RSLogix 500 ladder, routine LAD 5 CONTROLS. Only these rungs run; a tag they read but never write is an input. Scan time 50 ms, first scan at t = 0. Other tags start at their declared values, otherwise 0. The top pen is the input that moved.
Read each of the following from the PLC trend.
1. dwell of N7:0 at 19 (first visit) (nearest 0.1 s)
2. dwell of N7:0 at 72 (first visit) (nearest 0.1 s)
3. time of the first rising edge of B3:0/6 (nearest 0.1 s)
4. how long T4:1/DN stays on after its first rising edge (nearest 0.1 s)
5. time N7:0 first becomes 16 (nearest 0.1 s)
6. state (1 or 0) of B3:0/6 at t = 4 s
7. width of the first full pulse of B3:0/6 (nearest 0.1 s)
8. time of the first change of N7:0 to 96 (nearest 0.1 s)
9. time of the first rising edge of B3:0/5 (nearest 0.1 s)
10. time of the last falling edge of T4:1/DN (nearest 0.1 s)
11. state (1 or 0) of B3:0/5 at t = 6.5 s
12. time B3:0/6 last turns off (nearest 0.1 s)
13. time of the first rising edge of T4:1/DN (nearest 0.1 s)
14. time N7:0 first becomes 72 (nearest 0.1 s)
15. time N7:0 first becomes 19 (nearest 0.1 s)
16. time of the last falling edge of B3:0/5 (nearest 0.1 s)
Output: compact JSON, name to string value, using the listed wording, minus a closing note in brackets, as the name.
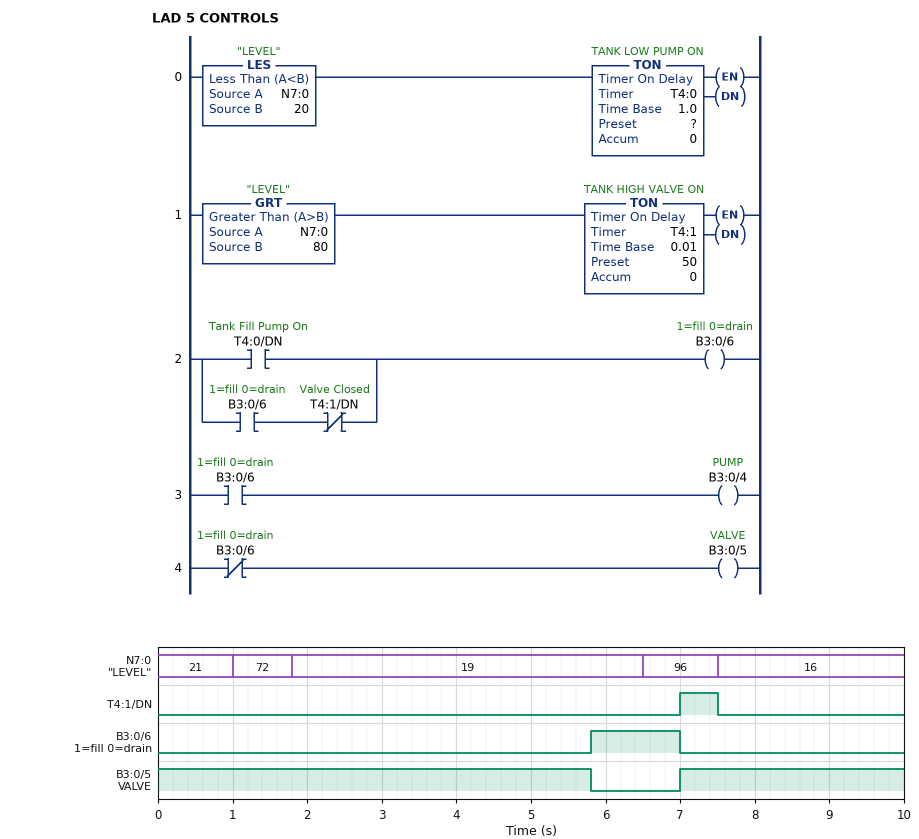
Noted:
{"dwell of N7:0 at 19 (first visit)": "4.7 s", "dwell of N7:0 at 72 (first visit)": "0.8 s", "time of the first rising edge of B3:0/6": "5.8 s", "how long T4:1/DN stays on after its first rising edge": "0.5 s", "time N7:0 first becomes 16": "7.5 s", "state (1 or 0) of B3:0/6 at t = 4 s": "0", "width of the first full pulse of B3:0/6": "1.2 s", "time of the first change of N7:0 to 96": "6.5 s", "time of the first rising edge of B3:0/5": "7.0 s", "time of the last falling edge of T4:1/DN": "7.5 s", "state (1 or 0) of B3:0/5 at t = 6.5 s": "0", "time B3:0/6 last turns off": "7.0 s", "time of the first rising edge of T4:1/DN": "7.0 s", "time N7:0 first becomes 72": "1.0 s", "time N7:0 first becomes 19": "1.8 s", "time of the last falling edge of B3:0/5": "5.8 s"}
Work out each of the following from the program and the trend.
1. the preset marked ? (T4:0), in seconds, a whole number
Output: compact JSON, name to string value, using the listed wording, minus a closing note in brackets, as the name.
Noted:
{"the preset marked ? (T4:0), in seconds, a whole number": "4 s"}
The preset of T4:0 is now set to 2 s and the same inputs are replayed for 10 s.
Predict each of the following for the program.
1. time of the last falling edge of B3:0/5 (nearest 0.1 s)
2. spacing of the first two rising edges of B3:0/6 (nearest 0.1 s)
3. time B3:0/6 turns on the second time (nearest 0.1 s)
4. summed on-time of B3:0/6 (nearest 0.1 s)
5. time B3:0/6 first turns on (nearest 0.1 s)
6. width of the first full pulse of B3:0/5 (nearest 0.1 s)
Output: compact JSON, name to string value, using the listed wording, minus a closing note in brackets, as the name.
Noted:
{"time of the last falling edge of B3:0/5": "9.5 s", "spacing of the first two rising edges of B3:0/6": "5.7 s", "time B3:0/6 turns on the second time": "9.5 s", "summed on-time of B3:0/6": "3.7 s", "time B3:0/6 first turns on": "3.8 s", "width of the first full pulse of B3:0/5": "2.5 s"}
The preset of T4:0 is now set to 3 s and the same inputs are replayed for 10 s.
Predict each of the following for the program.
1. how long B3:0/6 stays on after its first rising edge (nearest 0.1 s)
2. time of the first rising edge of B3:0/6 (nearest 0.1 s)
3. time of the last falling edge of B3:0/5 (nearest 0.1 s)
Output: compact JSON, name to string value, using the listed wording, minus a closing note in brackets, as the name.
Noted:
{"how long B3:0/6 stays on after its first rising edge": "2.2 s", "time of the first rising edge of B3:0/6": "4.8 s", "time of the last falling edge of B3:0/5": "4.8 s"}
